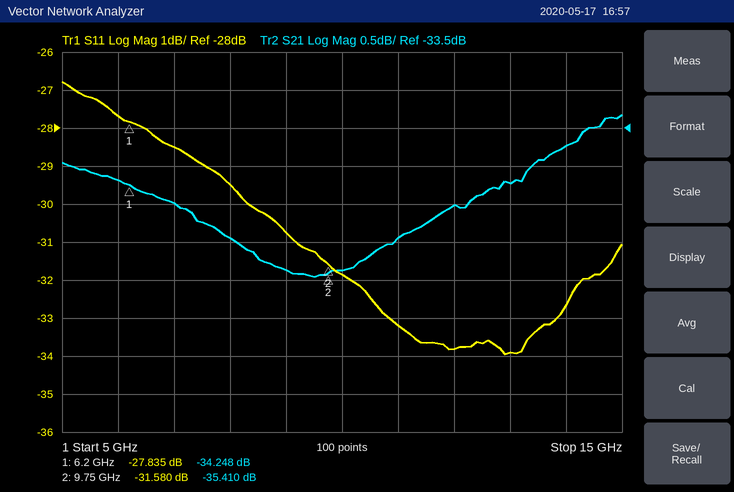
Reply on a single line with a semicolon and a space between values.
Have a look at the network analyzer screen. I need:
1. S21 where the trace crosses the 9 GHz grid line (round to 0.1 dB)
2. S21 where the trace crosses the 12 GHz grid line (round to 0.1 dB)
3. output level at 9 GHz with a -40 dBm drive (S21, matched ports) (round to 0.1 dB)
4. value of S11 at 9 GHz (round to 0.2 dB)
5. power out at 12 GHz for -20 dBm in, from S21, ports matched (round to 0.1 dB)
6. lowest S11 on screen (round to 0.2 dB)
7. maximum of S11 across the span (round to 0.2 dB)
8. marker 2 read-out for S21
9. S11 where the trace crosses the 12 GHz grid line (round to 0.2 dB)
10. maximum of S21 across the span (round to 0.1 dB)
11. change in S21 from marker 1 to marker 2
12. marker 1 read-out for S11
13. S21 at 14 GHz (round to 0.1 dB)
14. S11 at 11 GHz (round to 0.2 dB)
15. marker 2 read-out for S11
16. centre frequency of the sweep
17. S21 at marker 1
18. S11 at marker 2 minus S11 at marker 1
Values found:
-35.4 dB; -34.5 dB; -75.4 dBm; -30.8 dB; -54.5 dBm; -34.0 dB; -26.8 dB; -35.410 dB; -33.8 dB; -33.3 dB; -1.162 dB; -27.835 dB; -33.7 dB; -33.2 dB; -31.580 dB; 10 GHz; -34.248 dB; -3.745 dB
